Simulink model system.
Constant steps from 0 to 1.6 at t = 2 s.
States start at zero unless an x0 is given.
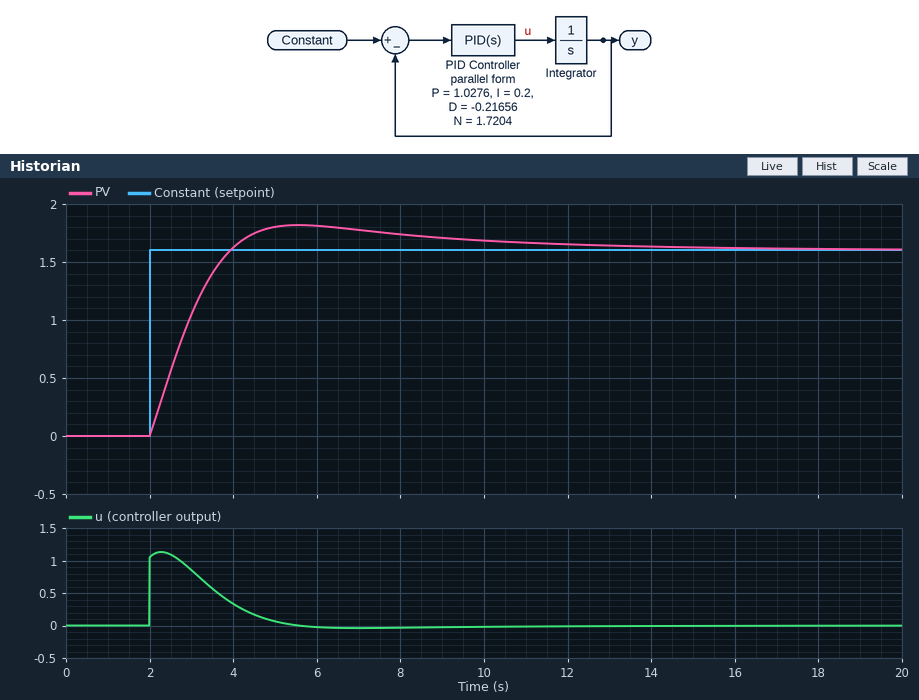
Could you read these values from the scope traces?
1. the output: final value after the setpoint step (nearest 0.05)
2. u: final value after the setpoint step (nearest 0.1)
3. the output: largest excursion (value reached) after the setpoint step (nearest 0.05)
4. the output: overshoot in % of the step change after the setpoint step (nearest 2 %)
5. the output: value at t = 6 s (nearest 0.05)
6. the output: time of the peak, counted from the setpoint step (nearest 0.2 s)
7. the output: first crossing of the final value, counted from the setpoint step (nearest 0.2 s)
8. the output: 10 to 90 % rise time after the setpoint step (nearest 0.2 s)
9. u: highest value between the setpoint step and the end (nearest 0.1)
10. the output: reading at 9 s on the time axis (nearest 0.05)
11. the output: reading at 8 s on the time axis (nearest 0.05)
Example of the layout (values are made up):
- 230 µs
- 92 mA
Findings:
- 1.60
- 0.0
- 1.80
- 14 %
- 1.80
- 3.6 s
- 2.0 s
- 1.4 s
- 1.1
- 1.70
- 1.75
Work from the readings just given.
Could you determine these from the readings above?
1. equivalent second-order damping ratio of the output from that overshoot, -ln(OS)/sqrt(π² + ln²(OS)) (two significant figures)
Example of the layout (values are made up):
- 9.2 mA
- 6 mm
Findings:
- 0.53
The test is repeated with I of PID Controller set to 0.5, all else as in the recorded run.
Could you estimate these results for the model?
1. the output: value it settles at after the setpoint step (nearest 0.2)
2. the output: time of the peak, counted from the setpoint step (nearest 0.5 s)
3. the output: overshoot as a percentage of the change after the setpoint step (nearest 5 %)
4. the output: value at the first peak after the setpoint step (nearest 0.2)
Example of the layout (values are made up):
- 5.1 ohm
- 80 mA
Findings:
- 1.6
- 3.0 s
- 25 %
- 2.0
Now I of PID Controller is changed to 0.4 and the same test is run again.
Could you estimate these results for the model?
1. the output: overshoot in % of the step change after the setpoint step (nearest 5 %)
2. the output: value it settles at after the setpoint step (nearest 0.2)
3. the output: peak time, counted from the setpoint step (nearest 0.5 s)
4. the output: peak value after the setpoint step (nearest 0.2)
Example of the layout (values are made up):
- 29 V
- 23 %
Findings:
- 20 %
- 1.6
- 3.0 s
- 2.0
